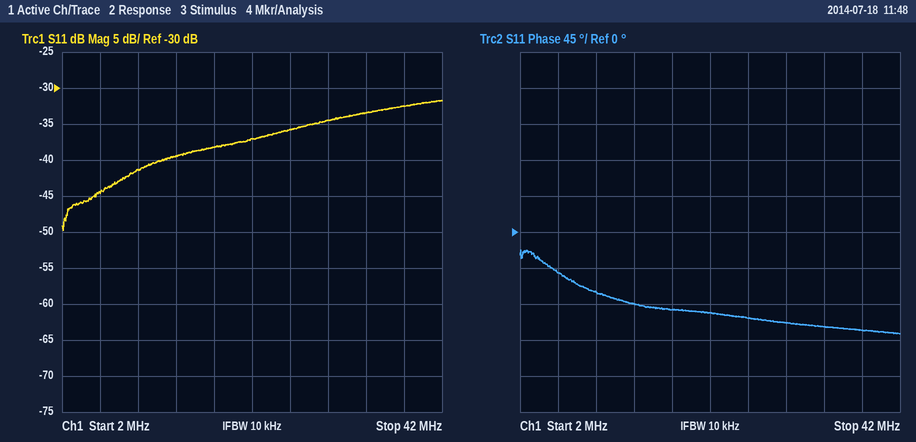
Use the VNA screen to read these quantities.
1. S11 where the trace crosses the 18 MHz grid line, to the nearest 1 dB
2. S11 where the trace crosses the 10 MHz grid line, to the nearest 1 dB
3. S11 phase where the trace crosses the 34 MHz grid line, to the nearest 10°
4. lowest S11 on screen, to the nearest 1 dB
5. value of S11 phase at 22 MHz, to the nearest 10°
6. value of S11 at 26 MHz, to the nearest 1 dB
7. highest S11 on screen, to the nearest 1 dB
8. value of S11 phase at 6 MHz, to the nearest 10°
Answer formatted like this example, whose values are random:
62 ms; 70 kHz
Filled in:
-38 dB; -41 dB; -120°; -50 dB; -100°; -36 dB; -32 dB; -50°
